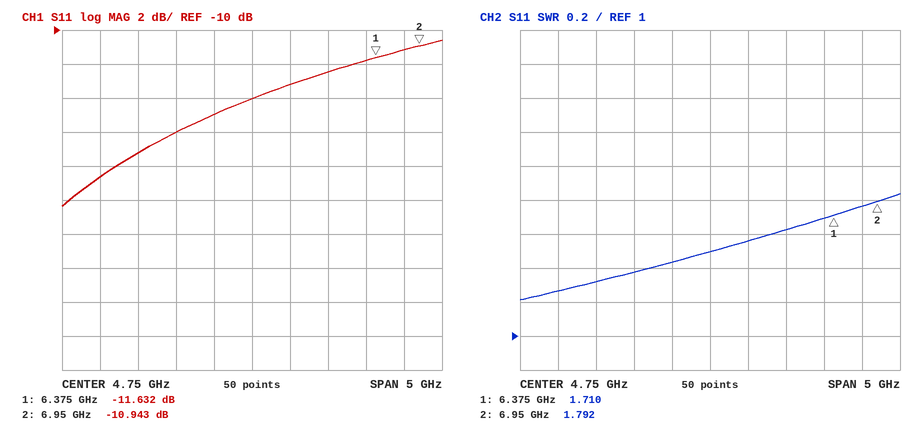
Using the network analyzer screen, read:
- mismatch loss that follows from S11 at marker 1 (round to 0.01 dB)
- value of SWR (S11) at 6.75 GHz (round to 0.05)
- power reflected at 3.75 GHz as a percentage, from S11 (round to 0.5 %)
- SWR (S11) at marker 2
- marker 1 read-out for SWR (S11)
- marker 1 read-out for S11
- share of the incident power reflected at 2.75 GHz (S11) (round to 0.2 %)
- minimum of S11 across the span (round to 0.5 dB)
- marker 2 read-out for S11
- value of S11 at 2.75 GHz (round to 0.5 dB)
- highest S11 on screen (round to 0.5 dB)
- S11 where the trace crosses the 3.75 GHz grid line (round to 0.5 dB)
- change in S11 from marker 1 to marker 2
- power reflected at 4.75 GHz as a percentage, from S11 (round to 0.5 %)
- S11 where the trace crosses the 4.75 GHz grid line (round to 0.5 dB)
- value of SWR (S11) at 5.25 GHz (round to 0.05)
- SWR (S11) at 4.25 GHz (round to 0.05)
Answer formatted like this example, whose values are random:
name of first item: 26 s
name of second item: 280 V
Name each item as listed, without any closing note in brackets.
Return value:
mismatch loss that follows from S11 at marker 1: 0.31 dB
value of SWR (S11) at 6.75 GHz: 1.75
power reflected at 3.75 GHz as a percentage, from S11: 2.5 %
SWR (S11) at marker 2: 1.792
marker 1 read-out for SWR: 1.710
marker 1 read-out for S11: -11.632 dB
share of the incident power reflected at 2.75 GHz (S11): 1.4 %
minimum of S11 across the span: -20.5 dB
marker 2 read-out for S11: -10.943 dB
value of S11 at 2.75 GHz: -18.5 dB
highest S11 on screen: -10.5 dB
S11 where the trace crosses the 3.75 GHz grid line: -16.0 dB
change in S11 from marker 1 to marker 2: 0.689 dB
power reflected at 4.75 GHz as a percentage, from S11: 4.0 %
S11 where the trace crosses the 4.75 GHz grid line: -14.0 dB
value of SWR (S11) at 5.25 GHz: 1.55
SWR (S11) at 4.25 GHz: 1.45
